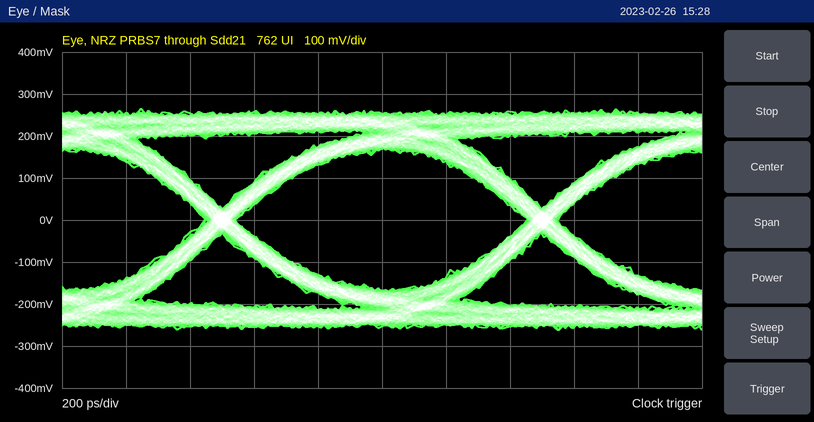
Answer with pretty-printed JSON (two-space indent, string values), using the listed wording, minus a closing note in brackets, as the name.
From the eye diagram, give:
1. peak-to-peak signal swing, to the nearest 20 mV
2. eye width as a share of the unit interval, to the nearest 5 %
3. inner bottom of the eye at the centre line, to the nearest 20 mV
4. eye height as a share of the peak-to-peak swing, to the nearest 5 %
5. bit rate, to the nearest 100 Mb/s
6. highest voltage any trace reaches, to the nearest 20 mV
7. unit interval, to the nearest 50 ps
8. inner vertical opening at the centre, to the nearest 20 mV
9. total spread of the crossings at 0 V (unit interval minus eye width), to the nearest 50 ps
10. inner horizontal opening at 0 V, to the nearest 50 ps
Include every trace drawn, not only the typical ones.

{
  "peak-to-peak signal swing, to the nearest 20 mV": "520 mV",
  "eye width as a share of the unit interval, to the nearest 5 %": "90 %",
  "inner bottom of the eye at the centre line, to the nearest 20 mV": "-160 mV",
  "eye height as a share of the peak-to-peak swing, to the nearest 5 %": "65 %",
  "bit rate, to the nearest 100 Mb/s": "1.0 Gb/s",
  "highest voltage any trace reaches, to the nearest 20 mV": "260 mV",
  "unit interval, to the nearest 50 ps": "1.00 ns",
  "inner vertical opening at the centre, to the nearest 20 mV": "340 mV",
  "total spread of the crossings at 0 V (unit interval minus eye width), to the nearest 50 ps": "100 ps",
  "inner horizontal opening at 0 V, to the nearest 50 ps": "900 ps"
}
